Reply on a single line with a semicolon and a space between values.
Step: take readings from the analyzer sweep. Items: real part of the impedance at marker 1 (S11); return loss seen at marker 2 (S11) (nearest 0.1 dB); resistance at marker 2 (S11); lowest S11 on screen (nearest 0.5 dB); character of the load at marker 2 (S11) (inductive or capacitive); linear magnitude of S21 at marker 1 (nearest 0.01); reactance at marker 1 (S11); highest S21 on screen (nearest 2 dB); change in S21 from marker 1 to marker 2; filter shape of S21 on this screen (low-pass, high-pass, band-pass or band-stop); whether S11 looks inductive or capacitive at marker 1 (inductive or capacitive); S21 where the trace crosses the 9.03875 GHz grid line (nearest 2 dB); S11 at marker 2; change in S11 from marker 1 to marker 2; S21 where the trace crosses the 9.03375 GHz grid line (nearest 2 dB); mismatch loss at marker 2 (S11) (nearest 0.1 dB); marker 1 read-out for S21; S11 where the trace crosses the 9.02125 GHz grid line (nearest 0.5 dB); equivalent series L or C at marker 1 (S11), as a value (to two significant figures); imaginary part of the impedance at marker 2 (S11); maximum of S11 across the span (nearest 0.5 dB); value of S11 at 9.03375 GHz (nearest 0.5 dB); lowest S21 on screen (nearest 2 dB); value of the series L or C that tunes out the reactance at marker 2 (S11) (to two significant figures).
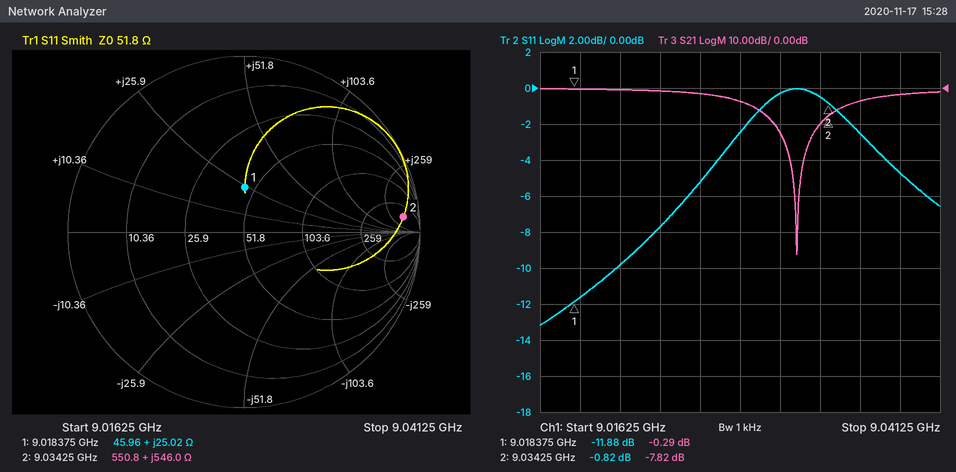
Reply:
45.96 Ω; 0.8 dB; 550.8 Ω; -13.0 dB; inductive; 0.97; +25.02 Ω; 0 dB; -7.53 dB; band-stop; inductive; -2 dB; -0.82 dB; 11.06 dB; -10 dB; 7.6 dB; -0.29 dB; -10.0 dB; 440 pH; +546.0 Ω; 0.0 dB; -0.5 dB; -46 dB; 32 fF
